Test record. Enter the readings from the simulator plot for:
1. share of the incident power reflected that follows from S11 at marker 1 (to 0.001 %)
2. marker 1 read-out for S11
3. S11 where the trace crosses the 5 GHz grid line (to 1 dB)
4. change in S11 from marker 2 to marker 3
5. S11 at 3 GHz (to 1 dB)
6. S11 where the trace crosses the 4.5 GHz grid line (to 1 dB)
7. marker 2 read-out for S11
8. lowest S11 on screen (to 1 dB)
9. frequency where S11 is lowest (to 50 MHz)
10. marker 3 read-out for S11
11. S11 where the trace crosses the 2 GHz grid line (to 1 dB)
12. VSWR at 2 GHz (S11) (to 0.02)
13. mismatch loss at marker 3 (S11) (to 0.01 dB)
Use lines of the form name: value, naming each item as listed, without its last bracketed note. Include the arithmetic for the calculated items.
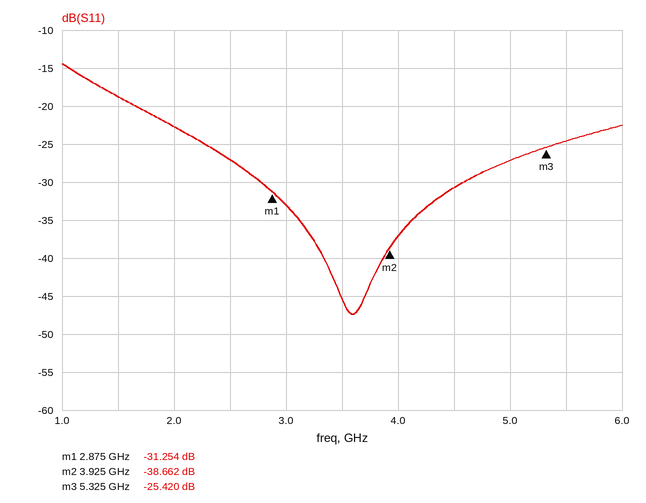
share of the incident power reflected that follows from S11 at marker 1: 10^(-31.254/10) ≈ 0.075 %
marker 1 read-out for S11: -31.254 dB
S11 where the trace crosses the 5 GHz grid line: -27 dB
change in S11 from marker 2 to marker 3: -25.42 − (-38.662) = 13.242 dB
S11 at 3 GHz: -33 dB
S11 where the trace crosses the 4.5 GHz grid line: -31 dB
marker 2 read-out for S11: -38.662 dB
lowest S11 on screen: -47 dB
frequency where S11 is lowest: 3.60 GHz
marker 3 read-out for S11: -25.420 dB
S11 where the trace crosses the 2 GHz grid line: -23 dB
VSWR at 2 GHz (S11): |Γ| = 10^(-23/20) = 0.0708; VSWR = (1 + 0.0708)/(1 − 0.0708) ≈ 1.15, so 1.16 to the nearest 0.02
mismatch loss at marker 3 (S11): −10 log10(1 − 10^(-25.42/10)) ≈ 0.01 dB
